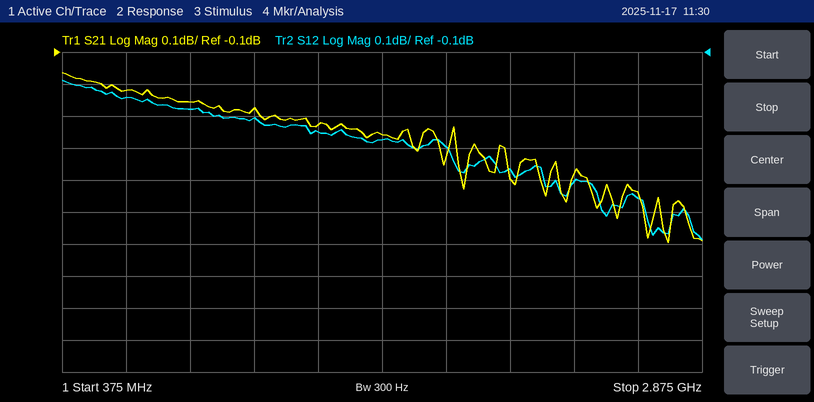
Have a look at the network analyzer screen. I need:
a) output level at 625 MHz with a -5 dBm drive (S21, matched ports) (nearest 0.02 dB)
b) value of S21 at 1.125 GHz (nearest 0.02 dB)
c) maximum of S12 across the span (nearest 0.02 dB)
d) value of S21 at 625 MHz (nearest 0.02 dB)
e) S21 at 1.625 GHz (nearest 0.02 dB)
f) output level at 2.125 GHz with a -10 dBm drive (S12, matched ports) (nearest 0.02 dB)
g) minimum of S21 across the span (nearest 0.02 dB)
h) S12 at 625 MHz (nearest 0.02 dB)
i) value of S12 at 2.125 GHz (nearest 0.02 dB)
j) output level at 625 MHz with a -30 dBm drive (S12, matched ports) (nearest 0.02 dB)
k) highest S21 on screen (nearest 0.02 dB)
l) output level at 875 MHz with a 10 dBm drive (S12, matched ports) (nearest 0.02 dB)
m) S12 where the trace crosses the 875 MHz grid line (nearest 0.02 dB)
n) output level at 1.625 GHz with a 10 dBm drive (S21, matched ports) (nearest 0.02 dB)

-5.22 dBm
-0.28 dB
-0.18 dB
-0.22 dB
-0.36 dB
-10.46 dBm
-0.70 dB
-0.24 dB
-0.46 dB
-30.24 dBm
-0.16 dB
9.72 dBm
-0.28 dB
9.64 dBm
